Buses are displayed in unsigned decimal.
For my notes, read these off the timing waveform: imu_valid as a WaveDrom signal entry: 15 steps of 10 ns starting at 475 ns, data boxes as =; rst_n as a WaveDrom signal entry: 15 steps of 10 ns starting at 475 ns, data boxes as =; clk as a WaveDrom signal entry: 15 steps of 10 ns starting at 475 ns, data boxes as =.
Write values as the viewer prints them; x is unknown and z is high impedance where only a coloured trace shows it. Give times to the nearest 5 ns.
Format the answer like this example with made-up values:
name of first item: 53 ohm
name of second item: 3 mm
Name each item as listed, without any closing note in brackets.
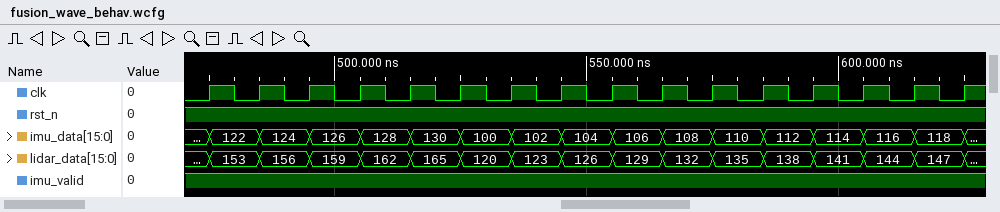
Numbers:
imu_valid as a WaveDrom signal entry: 15 steps of 10 ns starting at 475 ns, data boxes as =: {name: 'imu_valid', wave: '1..............'}
rst_n as a WaveDrom signal entry: 15 steps of 10 ns starting at 475 ns, data boxes as =: {name: 'rst_n', wave: '1..............'}
clk as a WaveDrom signal entry: 15 steps of 10 ns starting at 475 ns, data boxes as =: {name: 'clk', wave: 'p..............'}
